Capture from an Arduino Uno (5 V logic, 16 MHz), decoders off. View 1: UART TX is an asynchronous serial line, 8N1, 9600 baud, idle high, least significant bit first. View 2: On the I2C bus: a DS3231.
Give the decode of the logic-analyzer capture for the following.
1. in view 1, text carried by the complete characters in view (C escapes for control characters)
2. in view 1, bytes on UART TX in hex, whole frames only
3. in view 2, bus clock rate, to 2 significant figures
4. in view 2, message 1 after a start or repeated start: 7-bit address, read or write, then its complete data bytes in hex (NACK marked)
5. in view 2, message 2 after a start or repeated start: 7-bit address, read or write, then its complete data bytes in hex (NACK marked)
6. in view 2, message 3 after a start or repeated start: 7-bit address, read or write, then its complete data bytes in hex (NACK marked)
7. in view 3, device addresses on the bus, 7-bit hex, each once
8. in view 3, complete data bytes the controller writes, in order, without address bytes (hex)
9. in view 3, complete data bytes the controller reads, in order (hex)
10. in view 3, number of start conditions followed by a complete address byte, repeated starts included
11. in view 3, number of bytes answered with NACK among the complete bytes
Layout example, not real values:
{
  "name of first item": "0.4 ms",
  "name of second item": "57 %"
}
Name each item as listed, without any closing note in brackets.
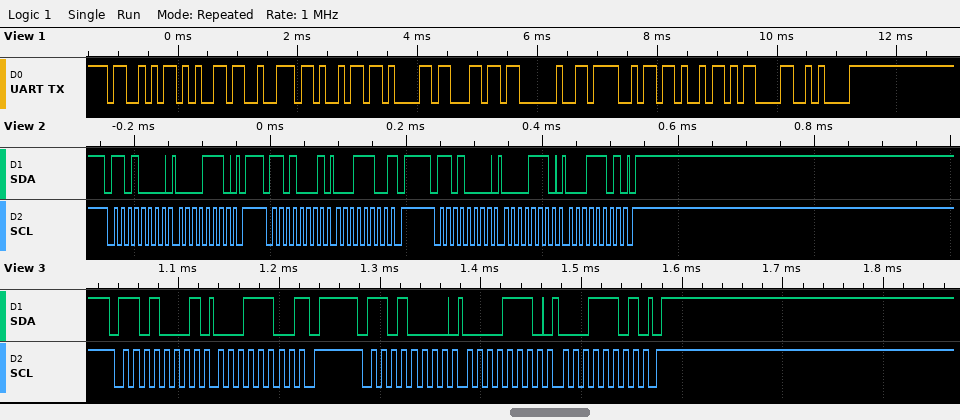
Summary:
{
  "in view 1, text carried by the complete characters in view": "\"Serial OK\\r\\n\"",
  "in view 1, bytes on UART TX in hex, whole frames only": "53 65 72 69 61 6C 20 4F 4B 0D 0A",
  "in view 2, bus clock rate, to 2 significant figures": "100 kHz",
  "in view 2, message 1 after a start or repeated start: 7-bit address, read or write, then its complete data bytes in hex": "0x68 write: 0E",
  "in view 2, message 2 after a start or repeated start: 7-bit address, read or write, then its complete data bytes in hex": "0x68 read: 1C NACK",
  "in view 2, message 3 after a start or repeated start: 7-bit address, read or write, then its complete data bytes in hex": "0x68 write: 0E 1D",
  "in view 3, device addresses on the bus, 7-bit hex, each once": "0x68",
  "in view 3, complete data bytes the controller writes, in order, without address bytes": "0E 1D",
  "in view 3, complete data bytes the controller reads, in order": "1C",
  "in view 3, number of start conditions followed by a complete address byte, repeated starts included": "2",
  "in view 3, number of bytes answered with NACK among the complete bytes": "1"
}
